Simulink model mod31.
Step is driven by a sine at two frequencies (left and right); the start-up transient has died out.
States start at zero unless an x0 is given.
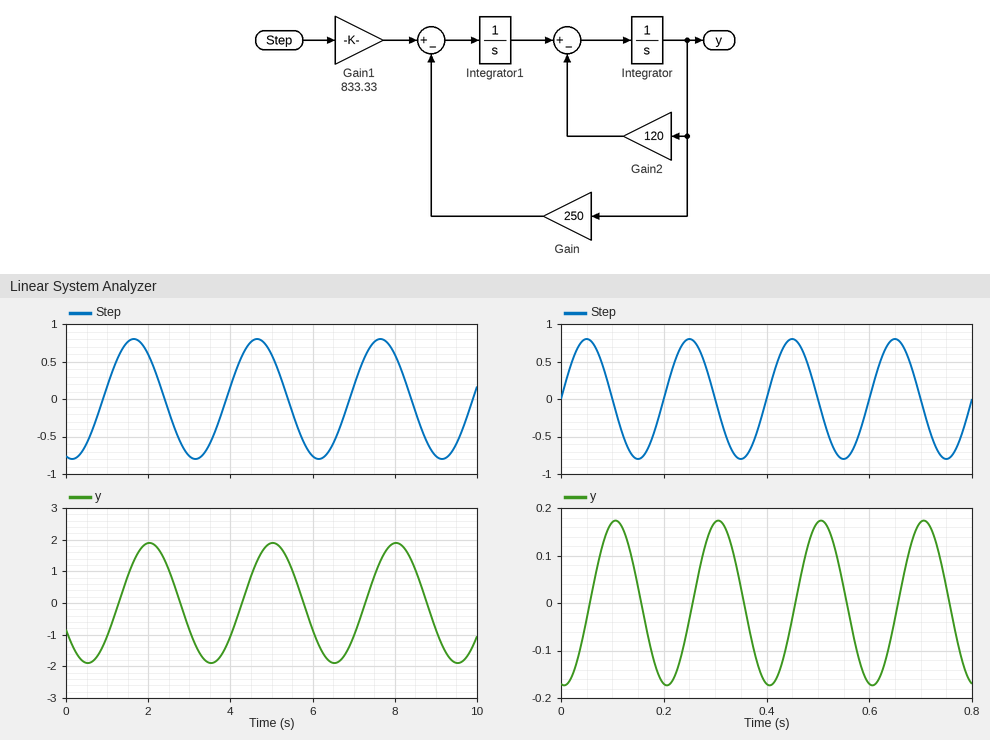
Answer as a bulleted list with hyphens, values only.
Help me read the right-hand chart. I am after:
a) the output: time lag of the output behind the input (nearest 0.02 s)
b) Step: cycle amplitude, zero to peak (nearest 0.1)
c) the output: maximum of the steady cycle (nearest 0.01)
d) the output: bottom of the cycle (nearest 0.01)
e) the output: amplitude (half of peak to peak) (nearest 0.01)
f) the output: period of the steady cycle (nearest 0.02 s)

- 0.06 s
- 0.8
- 0.17
- -0.17
- 0.17
- 0.20 s
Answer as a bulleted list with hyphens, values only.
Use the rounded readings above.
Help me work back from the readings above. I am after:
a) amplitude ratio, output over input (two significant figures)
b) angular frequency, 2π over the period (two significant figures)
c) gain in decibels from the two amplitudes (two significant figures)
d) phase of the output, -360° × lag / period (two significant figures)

- 0.21
- 31 rad/s
- -13 dB
- -110°
